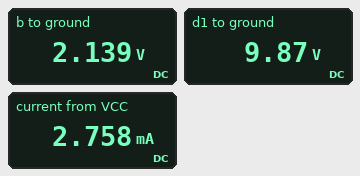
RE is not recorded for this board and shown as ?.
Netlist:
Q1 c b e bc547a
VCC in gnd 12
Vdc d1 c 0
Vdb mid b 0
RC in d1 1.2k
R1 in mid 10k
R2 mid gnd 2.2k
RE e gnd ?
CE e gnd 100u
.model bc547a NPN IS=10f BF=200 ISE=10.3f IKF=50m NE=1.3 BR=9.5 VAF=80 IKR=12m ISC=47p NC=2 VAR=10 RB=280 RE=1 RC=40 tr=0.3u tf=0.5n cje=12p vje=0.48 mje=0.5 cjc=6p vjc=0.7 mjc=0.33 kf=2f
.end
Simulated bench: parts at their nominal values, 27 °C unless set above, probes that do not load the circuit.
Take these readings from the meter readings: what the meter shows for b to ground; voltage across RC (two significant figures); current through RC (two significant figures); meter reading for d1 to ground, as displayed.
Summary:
2.139 V
2.1 V
1.8 mA
9.87 V
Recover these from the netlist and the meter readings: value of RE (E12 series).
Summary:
820 Ω
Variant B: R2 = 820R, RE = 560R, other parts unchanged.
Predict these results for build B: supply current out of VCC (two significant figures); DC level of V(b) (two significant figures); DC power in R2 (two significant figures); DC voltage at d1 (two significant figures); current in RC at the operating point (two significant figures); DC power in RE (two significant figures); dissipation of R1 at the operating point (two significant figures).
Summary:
1.6 mA
910 mV
1.0 mW
11 V
480 µA
130 µW
12 mW
